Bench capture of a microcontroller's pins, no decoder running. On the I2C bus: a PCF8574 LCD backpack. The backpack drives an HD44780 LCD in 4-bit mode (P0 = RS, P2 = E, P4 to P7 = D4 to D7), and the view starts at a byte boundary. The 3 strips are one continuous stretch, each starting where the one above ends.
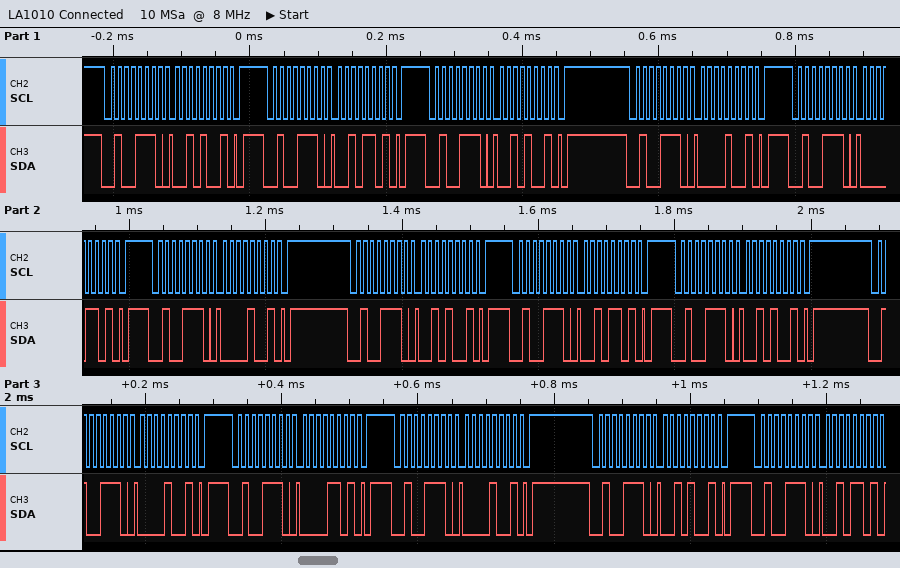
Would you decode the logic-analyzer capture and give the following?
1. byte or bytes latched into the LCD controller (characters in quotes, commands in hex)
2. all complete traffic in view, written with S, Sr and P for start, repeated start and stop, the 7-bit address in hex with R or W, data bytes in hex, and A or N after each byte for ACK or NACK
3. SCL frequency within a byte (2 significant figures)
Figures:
' ' ' '
S 27W A 29 A P S 27W A 2D A P S 27W A 29 A P S 27W A 09 A P S 27W A 0D A P S 27W A 09 A P S 27W A 29 A P S 27W A 2D A P S 27W A 29 A P S 27W A 09 A P S 27W A 0D A P S 27W A 09 A P S 27W A 29 A P S 27W A 2D A
100 kHz
